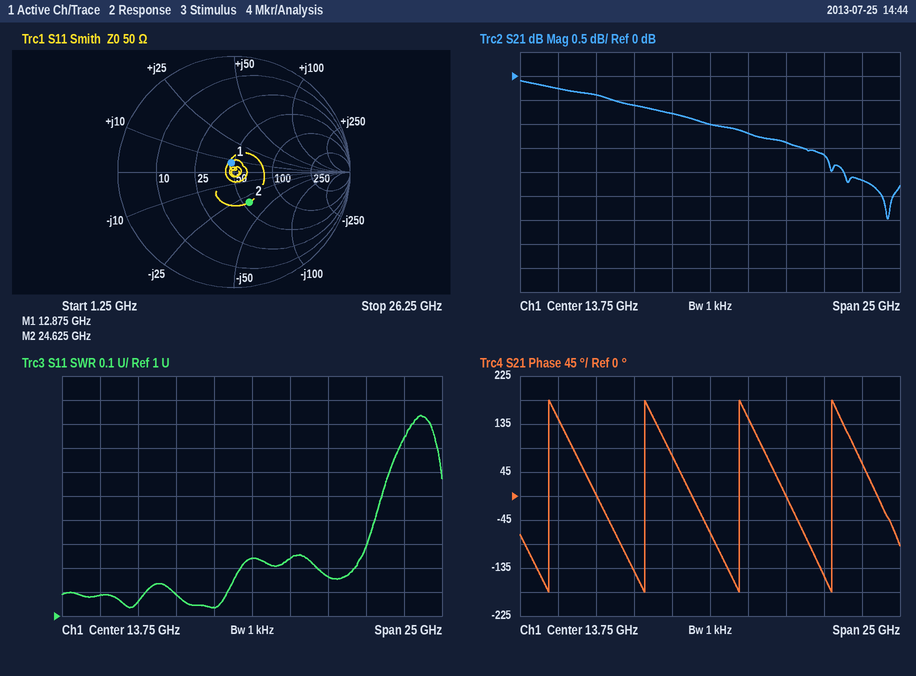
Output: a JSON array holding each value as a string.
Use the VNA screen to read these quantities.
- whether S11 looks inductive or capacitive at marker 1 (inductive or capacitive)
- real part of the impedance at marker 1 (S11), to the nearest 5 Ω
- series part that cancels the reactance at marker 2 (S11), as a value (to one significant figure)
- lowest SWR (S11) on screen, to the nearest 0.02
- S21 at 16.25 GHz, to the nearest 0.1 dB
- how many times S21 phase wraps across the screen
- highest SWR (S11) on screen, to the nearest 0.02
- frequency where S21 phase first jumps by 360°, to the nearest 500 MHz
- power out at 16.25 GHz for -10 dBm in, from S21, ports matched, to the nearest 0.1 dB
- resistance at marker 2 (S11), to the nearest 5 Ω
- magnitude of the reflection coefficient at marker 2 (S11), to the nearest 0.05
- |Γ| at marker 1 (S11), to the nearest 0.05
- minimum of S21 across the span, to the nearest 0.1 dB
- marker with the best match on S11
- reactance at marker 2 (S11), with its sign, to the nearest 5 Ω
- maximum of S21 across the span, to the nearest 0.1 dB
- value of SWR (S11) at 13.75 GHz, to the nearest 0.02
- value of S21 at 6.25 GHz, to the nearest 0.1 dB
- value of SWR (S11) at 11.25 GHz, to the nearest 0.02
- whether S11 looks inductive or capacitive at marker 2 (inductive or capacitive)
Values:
["inductive", "45 Ω", "200 pH", "1.04", "-1.2 dB", "4", "1.84", "3.0 GHz", "-11.2 dBm", "55 Ω", "0.30", "0.10", "-3.0 dB", "marker 1", "-30 Ω", "-0.1 dB", "1.24", "-0.4 dB", "1.04", "capacitive"]
